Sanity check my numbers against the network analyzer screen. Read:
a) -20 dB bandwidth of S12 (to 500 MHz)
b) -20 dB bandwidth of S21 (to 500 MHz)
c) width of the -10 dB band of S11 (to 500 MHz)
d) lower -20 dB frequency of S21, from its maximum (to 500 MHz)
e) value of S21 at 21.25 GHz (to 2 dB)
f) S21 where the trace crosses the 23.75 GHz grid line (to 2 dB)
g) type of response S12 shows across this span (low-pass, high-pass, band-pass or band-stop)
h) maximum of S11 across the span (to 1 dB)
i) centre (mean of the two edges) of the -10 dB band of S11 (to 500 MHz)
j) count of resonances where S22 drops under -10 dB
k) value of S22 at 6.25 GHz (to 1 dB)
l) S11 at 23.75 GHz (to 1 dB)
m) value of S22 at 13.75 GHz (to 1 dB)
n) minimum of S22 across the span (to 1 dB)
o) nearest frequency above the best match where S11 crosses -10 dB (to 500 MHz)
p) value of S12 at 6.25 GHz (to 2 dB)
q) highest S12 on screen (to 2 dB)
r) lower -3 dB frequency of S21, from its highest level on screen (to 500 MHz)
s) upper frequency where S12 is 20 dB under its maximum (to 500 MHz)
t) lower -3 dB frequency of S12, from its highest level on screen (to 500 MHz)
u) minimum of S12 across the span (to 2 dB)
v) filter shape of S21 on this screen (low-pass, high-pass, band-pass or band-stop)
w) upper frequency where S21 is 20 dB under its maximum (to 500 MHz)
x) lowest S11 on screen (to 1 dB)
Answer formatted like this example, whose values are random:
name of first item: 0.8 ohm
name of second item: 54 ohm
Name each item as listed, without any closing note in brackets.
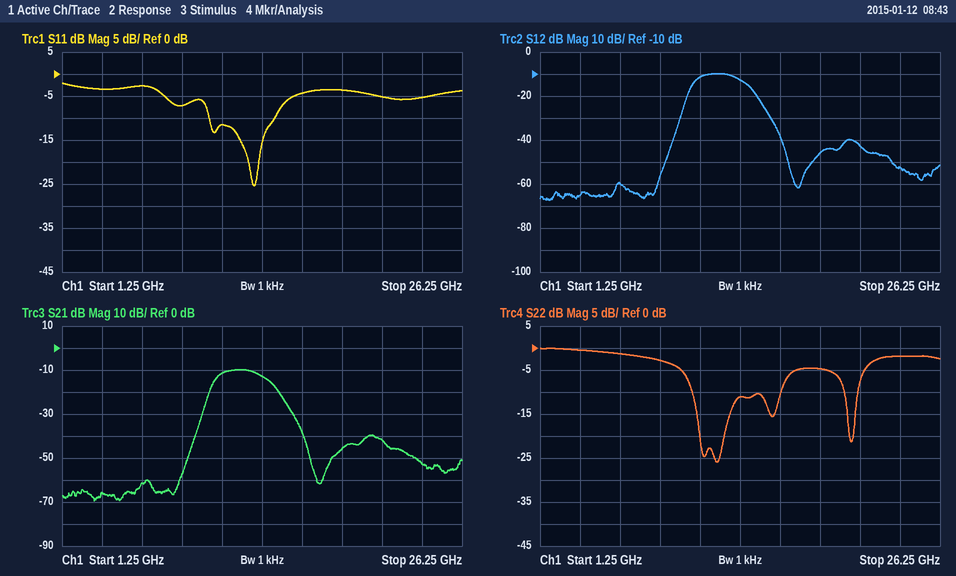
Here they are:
-20 dB bandwidth of S12: 5.5 GHz
-20 dB bandwidth of S21: 5.5 GHz
width of the -10 dB band of S11: 4.0 GHz
lower -20 dB frequency of S21, from its maximum: 10.0 GHz
value of S21 at 21.25 GHz: -42 dB
S21 where the trace crosses the 23.75 GHz grid line: -52 dB
type of response S12 shows across this span: band-pass
maximum of S11 across the span: -2 dB
centre (mean of the two edges) of the -10 dB band of S11: 12.5 GHz
count of resonances where S22 drops under -10 dB: 3
value of S22 at 6.25 GHz: -1 dB
S11 at 23.75 GHz: -5 dB
value of S22 at 13.75 GHz: -11 dB
minimum of S22 across the span: -26 dB
nearest frequency above the best match where S11 crosses -10 dB: 14.5 GHz
value of S12 at 6.25 GHz: -60 dB
highest S12 on screen: -10 dB
lower -3 dB frequency of S21, from its highest level on screen: 11.0 GHz
upper frequency where S12 is 20 dB under its maximum: 15.5 GHz
lower -3 dB frequency of S12, from its highest level on screen: 11.0 GHz
minimum of S12 across the span: -68 dB
filter shape of S21 on this screen: band-pass
upper frequency where S21 is 20 dB under its maximum: 15.5 GHz
lowest S11 on screen: -25 dB
